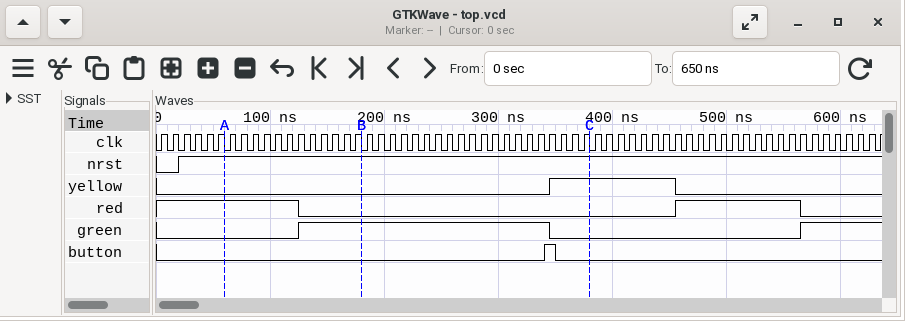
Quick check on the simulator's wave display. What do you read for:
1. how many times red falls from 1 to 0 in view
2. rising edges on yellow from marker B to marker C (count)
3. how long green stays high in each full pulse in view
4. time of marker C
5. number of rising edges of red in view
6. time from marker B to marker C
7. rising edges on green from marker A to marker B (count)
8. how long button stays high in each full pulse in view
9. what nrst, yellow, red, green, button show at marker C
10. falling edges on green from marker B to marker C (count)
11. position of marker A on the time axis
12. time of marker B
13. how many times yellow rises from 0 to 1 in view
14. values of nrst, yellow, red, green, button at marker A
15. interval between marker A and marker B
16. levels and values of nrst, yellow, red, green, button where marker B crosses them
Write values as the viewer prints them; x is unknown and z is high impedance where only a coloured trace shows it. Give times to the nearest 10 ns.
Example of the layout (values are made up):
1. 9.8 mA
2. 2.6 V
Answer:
1. 2
2. 1
3. 220 ns
4. 380 ns
5. 1
6. 200 ns
7. 1
8. 10 ns
9. nrst=1, yellow=1, red=0, green=0, button=0
10. 1
11. 60 ns
12. 180 ns
13. 1
14. nrst=1, yellow=0, red=1, green=0, button=0
15. 120 ns
16. nrst=1, yellow=0, red=0, green=1, button=0
